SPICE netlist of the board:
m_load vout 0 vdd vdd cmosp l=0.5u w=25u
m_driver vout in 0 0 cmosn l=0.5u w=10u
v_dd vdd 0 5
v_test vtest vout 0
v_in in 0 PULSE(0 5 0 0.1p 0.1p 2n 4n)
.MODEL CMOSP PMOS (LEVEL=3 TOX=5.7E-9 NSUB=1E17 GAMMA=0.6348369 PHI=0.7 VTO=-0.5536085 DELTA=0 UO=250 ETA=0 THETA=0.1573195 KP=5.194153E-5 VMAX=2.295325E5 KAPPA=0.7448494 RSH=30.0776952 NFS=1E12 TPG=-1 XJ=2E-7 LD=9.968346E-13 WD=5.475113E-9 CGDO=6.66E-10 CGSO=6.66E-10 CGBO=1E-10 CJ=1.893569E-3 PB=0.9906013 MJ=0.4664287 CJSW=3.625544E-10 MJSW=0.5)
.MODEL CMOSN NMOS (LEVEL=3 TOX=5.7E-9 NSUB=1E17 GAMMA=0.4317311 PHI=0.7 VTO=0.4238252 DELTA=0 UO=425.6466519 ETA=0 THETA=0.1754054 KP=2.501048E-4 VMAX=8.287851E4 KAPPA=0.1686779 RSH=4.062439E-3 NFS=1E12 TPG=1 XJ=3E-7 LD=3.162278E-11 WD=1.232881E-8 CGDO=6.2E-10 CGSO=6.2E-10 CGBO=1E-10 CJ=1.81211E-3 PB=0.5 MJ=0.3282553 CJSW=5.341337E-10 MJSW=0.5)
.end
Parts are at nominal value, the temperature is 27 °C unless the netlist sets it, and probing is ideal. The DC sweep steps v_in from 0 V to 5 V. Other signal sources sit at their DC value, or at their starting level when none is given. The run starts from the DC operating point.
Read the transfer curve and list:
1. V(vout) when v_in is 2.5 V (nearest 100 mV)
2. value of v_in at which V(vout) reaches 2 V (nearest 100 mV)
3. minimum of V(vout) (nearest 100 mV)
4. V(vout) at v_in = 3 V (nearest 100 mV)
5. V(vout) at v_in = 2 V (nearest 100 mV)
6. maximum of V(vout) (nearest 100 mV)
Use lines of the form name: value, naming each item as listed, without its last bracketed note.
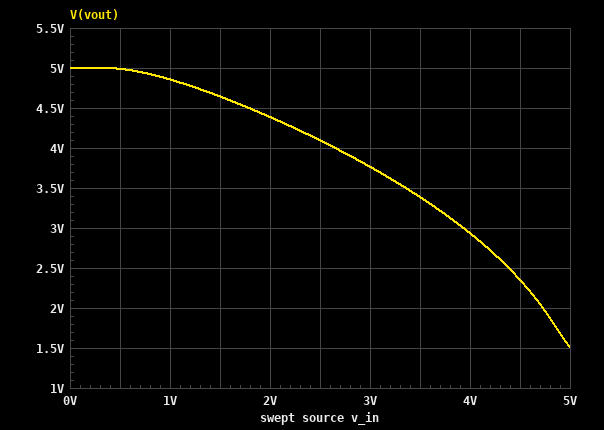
V(vout) when v_in is 2.5 V: 4.1 V
value of v_in at which V(vout) reaches 2 V: 4.7 V
minimum of V(vout): 1.5 V
V(vout) at v_in = 3 V: 3.8 V
V(vout) at v_in = 2 V: 4.4 V
maximum of V(vout): 5.0 V
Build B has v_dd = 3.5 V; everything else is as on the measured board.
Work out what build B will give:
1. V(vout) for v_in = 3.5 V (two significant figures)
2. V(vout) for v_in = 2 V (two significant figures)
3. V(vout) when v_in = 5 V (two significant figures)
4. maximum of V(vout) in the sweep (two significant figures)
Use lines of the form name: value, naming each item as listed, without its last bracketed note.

V(vout) for v_in = 3.5 V: 890 mV
V(vout) for v_in = 2 V: 2.7 V
V(vout) when v_in = 5 V: 520 mV
maximum of V(vout) in the sweep: 3.5 V
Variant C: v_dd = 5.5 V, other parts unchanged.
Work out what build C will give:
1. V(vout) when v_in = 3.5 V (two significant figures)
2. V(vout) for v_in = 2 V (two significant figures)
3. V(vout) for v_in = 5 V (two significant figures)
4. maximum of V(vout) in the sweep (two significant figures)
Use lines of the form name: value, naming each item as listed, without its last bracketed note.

V(vout) when v_in = 3.5 V: 4.0 V
V(vout) for v_in = 2 V: 4.9 V
V(vout) for v_in = 5 V: 2.6 V
maximum of V(vout) in the sweep: 5.5 V
